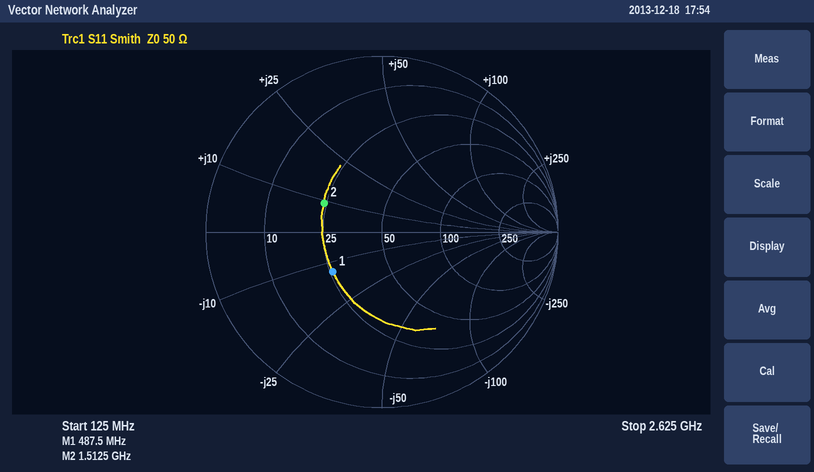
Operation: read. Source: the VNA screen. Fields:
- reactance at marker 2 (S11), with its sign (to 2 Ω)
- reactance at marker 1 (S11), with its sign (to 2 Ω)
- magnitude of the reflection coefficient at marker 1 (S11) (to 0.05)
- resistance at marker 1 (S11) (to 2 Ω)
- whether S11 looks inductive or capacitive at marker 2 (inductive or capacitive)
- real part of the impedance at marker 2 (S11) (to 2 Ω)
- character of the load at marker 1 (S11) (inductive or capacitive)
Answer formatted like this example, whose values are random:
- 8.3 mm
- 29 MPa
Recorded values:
- +10 Ω
- -14 Ω
- 0.35
- 26 Ω
- inductive
- 24 Ω
- capacitive
